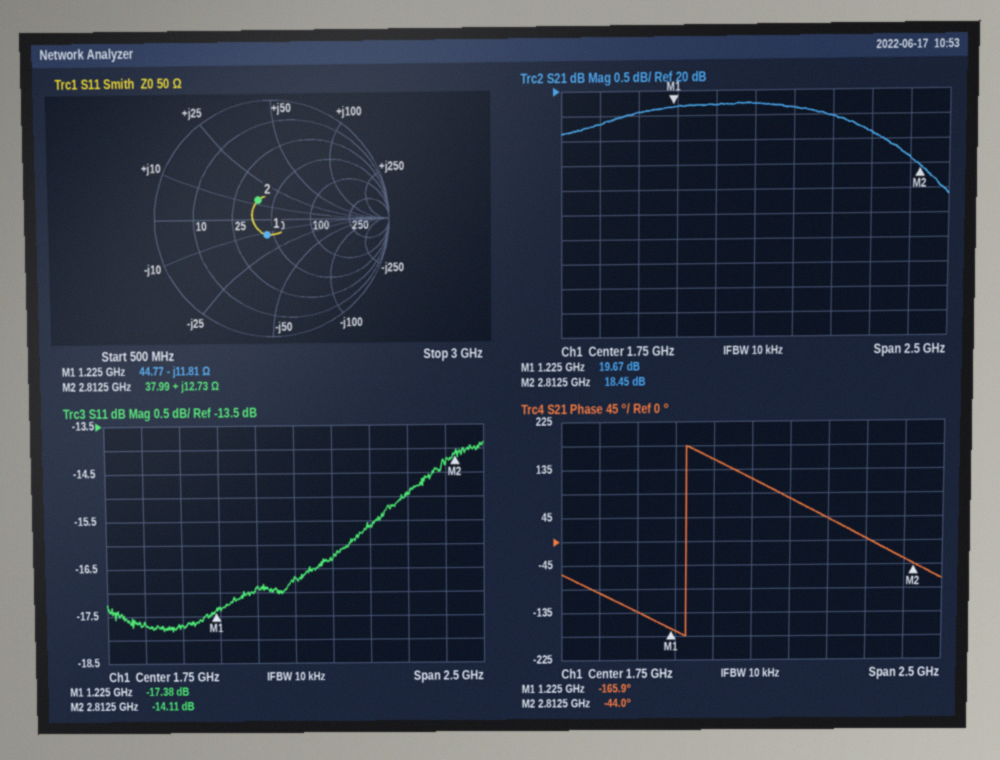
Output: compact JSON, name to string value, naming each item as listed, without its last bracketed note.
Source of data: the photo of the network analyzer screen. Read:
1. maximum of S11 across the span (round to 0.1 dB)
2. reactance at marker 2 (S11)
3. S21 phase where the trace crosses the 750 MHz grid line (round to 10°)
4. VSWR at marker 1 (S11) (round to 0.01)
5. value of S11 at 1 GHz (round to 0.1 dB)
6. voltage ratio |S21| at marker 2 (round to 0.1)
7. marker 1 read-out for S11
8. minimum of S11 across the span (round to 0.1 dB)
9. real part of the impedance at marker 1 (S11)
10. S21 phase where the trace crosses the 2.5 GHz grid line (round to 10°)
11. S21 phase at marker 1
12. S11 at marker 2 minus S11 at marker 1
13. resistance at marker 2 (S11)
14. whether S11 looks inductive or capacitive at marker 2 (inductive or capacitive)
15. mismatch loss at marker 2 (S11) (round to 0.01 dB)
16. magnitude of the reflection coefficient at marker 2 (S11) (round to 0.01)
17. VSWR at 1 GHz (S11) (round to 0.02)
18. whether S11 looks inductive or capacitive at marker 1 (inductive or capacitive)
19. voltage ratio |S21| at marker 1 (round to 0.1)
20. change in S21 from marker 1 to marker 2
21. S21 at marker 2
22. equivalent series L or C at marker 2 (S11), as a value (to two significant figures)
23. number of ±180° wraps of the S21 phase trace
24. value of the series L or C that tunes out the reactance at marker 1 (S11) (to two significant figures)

{"maximum of S11 across the span": "-13.9 dB", "reactance at marker 2": "+12.73 Ω", "S21 phase where the trace crosses the 750 MHz grid line": "-100°", "VSWR at marker 1 (S11)": "1.31", "value of S11 at 1 GHz": "-17.7 dB", "voltage ratio |S21| at marker 2": "8.4", "marker 1 read-out for S11": "-17.38 dB", "minimum of S11 across the span": "-17.8 dB", "real part of the impedance at marker 1": "44.77 Ω", "S21 phase where the trace crosses the 2.5 GHz grid line": "0°", "S21 phase at marker 1": "-165.9°", "S11 at marker 2 minus S11 at marker 1": "3.27 dB", "resistance at marker 2": "37.99 Ω", "whether S11 looks inductive or capacitive at marker 2": "inductive", "mismatch loss at marker 2 (S11)": "0.17 dB", "magnitude of the reflection coefficient at marker 2 (S11)": "0.20", "VSWR at 1 GHz (S11)": "1.30", "whether S11 looks inductive or capacitive at marker 1": "capacitive", "voltage ratio |S21| at marker 1": "9.6", "change in S21 from marker 1 to marker 2": "-1.22 dB", "S21 at marker 2": "18.45 dB", "equivalent series L or C at marker 2 (S11), as a value": "720 pH", "number of ±180° wraps of the S21 phase trace": "1", "value of the series L or C that tunes out the reactance at marker 1 (S11)": "1.5 nH"}
